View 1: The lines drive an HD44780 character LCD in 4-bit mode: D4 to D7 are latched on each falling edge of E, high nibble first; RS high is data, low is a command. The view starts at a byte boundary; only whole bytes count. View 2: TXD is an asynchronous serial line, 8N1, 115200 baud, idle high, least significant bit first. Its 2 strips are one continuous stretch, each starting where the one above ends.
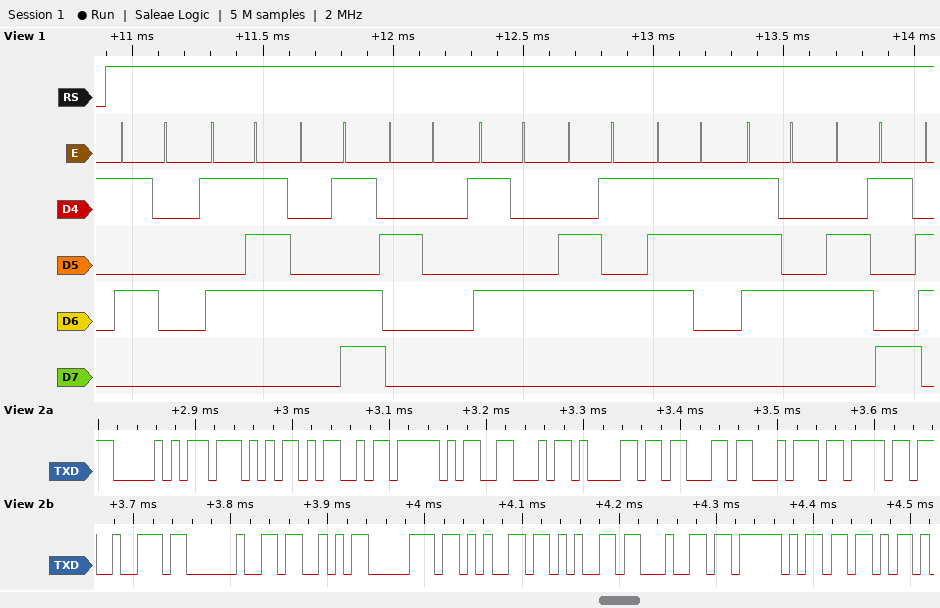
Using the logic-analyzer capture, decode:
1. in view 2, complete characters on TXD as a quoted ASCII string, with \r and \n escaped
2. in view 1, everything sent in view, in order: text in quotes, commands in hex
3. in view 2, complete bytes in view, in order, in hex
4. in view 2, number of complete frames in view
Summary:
"PWM_Factor Speed_["
"PWM Testi"
0x50 0x57 0x4D 0x5F 0x46 0x61 0x63 0x74 0x6F 0x72 0x20 0x53 0x70 0x65 0x65 0x64 0x5F 0x5B
18
